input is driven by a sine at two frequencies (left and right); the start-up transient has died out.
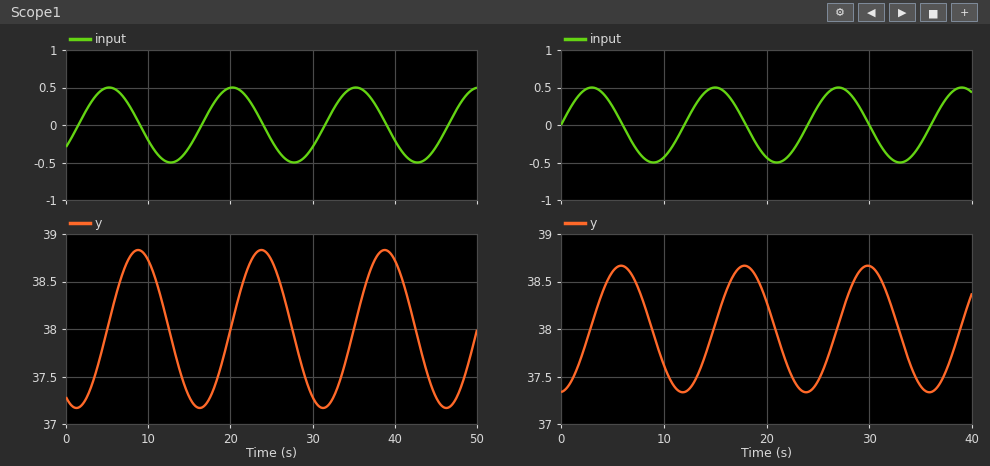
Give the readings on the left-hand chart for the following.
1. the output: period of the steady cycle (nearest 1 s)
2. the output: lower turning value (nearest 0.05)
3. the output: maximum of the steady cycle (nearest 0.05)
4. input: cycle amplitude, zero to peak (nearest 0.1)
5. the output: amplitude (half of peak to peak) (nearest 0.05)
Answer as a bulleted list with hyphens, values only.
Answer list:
- 15 s
- 37.15
- 38.85
- 0.5
- 0.85
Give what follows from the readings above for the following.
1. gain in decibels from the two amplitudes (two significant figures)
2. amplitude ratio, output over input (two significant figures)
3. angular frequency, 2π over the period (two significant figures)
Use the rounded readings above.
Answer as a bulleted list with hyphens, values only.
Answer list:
- 4.6 dB
- 1.7
- 0.42 rad/s
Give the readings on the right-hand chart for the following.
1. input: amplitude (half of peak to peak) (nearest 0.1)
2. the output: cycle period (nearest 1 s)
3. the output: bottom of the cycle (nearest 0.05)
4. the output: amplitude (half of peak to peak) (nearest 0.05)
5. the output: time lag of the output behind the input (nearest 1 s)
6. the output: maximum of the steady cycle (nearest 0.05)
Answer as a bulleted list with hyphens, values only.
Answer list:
- 0.5
- 12 s
- 37.35
- 0.65
- 3 s
- 38.65
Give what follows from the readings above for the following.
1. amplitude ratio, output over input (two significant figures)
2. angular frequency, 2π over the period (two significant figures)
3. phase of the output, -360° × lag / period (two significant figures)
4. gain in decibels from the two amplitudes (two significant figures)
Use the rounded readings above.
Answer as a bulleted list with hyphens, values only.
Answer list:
- 1.3
- 0.52 rad/s
- -90°
- 2.3 dB
